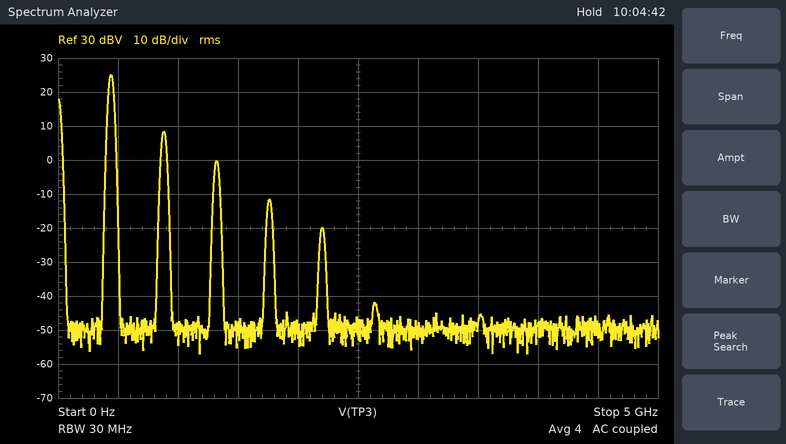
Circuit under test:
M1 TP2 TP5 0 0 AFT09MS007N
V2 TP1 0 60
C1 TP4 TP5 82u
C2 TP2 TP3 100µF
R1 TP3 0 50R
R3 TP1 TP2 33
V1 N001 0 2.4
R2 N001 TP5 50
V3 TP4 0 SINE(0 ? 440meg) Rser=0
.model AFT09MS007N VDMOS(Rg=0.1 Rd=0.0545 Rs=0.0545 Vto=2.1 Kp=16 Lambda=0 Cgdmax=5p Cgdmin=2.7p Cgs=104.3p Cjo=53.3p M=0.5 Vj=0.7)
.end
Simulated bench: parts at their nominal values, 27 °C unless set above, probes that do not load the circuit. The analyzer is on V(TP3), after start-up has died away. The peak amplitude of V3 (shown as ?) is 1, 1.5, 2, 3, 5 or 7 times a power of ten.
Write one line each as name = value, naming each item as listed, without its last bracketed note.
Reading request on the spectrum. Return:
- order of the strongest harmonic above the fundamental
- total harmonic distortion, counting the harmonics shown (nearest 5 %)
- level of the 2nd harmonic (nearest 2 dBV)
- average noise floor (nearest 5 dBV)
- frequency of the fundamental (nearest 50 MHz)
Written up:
order of the strongest harmonic above the fundamental = 2
total harmonic distortion, counting the harmonics shown = 15 %
level of the 2nd harmonic = 8 dBV
average noise floor = -50 dBV
frequency of the fundamental = 450 MHz
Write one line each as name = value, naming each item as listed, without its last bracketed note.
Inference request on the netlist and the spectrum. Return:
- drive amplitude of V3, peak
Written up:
drive amplitude of V3, peak = 500 mV
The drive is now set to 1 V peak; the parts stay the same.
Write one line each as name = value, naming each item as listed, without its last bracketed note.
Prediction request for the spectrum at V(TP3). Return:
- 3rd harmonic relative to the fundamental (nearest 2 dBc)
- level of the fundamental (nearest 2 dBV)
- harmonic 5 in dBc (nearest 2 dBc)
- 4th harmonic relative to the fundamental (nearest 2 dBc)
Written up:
3rd harmonic relative to the fundamental = -14 dBc
level of the fundamental = 26 dBV
harmonic 5 in dBc = -30 dBc
4th harmonic relative to the fundamental = -26 dBc
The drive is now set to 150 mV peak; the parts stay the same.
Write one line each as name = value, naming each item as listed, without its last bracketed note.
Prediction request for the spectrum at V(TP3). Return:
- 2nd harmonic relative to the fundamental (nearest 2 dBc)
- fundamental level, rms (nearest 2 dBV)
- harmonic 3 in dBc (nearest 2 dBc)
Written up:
2nd harmonic relative to the fundamental = -24 dBc
fundamental level, rms = 16 dBV
harmonic 3 in dBc = -46 dBc
